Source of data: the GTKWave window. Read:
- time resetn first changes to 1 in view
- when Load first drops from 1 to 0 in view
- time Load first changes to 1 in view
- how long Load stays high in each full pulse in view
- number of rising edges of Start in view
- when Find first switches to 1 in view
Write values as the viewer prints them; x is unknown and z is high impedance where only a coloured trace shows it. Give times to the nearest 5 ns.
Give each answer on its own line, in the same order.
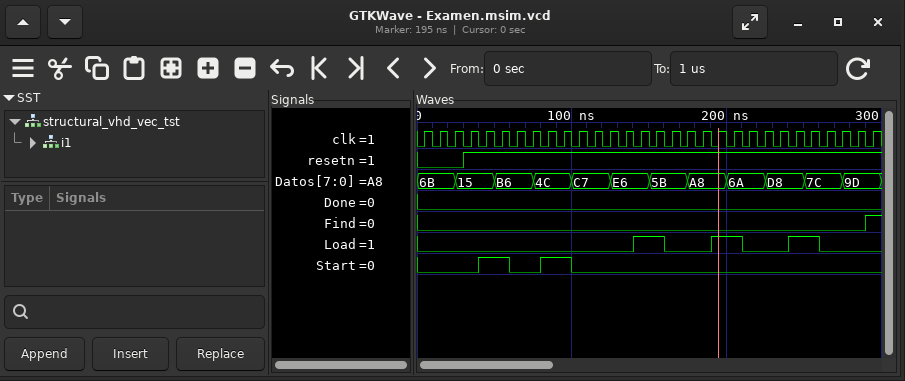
30 ns
160 ns
140 ns
20 ns, 20 ns, 20 ns
2
290 ns
